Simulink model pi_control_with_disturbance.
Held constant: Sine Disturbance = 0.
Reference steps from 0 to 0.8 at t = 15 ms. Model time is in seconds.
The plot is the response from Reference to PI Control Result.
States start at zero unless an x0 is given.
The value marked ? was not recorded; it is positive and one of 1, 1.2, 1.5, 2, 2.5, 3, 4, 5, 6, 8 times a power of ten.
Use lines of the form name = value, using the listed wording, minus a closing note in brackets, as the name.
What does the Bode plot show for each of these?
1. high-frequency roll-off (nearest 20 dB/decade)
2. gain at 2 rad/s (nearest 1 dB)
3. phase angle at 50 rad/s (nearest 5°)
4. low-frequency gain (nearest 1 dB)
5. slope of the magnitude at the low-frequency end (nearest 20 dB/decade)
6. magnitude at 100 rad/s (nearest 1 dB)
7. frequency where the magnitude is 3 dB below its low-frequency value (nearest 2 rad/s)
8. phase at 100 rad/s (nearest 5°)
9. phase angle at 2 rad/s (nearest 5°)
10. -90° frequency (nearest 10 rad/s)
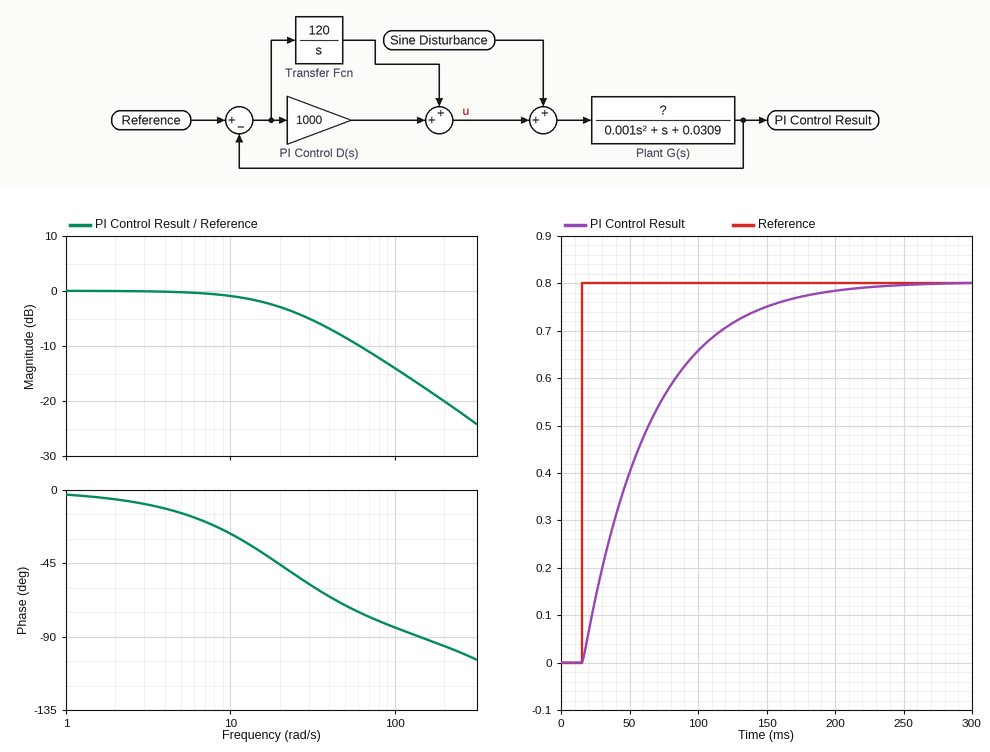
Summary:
high-frequency roll-off = -20 dB/decade
gain at 2 rad/s = 0 dB
phase angle at 50 rad/s = -70°
low-frequency gain = 0 dB
slope of the magnitude at the low-frequency end = 0 dB/decade
magnitude at 100 rad/s = -14 dB
frequency where the magnitude is 3 dB below its low-frequency value = 20 rad/s
phase at 100 rad/s = -85°
phase angle at 2 rad/s = -5°
-90° frequency = 140 rad/s
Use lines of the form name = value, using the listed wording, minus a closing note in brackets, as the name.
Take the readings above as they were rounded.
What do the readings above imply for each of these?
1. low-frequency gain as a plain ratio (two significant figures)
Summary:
low-frequency gain as a plain ratio = 1.0
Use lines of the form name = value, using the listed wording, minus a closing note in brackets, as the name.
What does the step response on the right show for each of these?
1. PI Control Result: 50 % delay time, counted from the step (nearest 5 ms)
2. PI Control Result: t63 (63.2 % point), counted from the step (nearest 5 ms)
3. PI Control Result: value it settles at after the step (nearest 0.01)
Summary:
PI Control Result: 50 % delay time, counted from the step = 35 ms
PI Control Result: t63 (63.2 % point), counted from the step = 50 ms
PI Control Result: value it settles at after the step = 0.80
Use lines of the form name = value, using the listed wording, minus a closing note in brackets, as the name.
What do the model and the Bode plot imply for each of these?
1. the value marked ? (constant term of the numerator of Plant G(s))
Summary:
the value marked ? (constant term of the numerator of Plant G(s)) = 0.02
